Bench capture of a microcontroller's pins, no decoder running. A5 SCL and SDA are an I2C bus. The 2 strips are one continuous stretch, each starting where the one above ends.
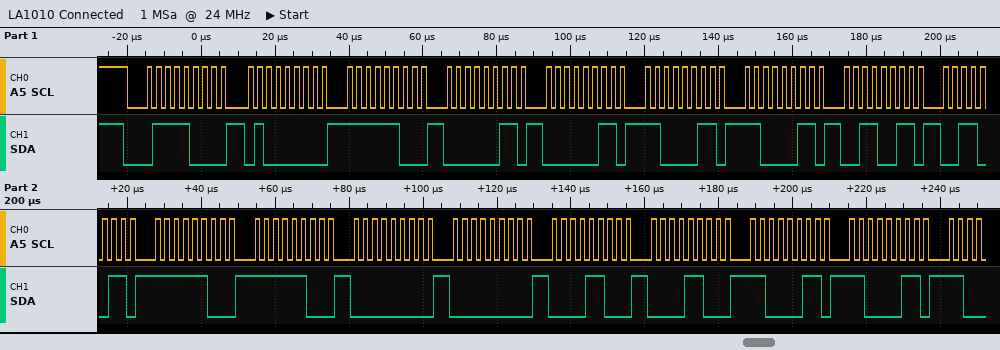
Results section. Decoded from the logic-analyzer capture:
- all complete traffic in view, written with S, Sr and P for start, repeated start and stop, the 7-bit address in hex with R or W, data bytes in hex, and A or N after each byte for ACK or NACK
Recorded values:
S 3CW A 40 A FC A 03 A 03 A C3 A C3 A 33 A 33 A FC A FC A 00 A 00 A 0C A 0C A C3 A C3 A
